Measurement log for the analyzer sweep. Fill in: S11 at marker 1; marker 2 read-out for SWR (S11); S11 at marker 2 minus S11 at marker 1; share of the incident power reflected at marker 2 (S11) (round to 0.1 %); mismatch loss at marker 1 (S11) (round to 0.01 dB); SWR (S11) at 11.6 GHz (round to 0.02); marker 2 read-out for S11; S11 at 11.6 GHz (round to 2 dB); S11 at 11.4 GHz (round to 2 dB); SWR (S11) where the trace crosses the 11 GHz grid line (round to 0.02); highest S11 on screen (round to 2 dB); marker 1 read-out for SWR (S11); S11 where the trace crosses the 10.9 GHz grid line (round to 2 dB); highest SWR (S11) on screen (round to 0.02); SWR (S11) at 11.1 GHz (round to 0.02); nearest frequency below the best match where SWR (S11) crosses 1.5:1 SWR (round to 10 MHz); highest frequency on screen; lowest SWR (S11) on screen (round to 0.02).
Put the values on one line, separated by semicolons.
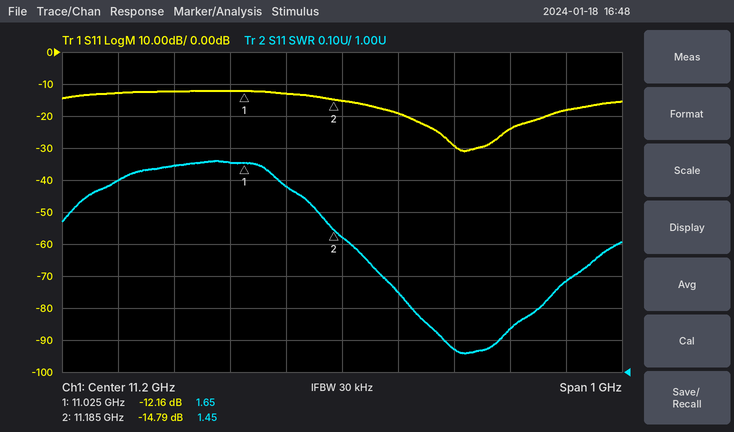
-12.16 dB; 1.45; -2.63 dB; 3.3 %; 0.27 dB; 1.28; -14.79 dB; -18 dB; -30 dB; 1.66; -12 dB; 1.65; -12 dB; 1.66; 1.58; 11.16 GHz; 11.7 GHz; 1.06
